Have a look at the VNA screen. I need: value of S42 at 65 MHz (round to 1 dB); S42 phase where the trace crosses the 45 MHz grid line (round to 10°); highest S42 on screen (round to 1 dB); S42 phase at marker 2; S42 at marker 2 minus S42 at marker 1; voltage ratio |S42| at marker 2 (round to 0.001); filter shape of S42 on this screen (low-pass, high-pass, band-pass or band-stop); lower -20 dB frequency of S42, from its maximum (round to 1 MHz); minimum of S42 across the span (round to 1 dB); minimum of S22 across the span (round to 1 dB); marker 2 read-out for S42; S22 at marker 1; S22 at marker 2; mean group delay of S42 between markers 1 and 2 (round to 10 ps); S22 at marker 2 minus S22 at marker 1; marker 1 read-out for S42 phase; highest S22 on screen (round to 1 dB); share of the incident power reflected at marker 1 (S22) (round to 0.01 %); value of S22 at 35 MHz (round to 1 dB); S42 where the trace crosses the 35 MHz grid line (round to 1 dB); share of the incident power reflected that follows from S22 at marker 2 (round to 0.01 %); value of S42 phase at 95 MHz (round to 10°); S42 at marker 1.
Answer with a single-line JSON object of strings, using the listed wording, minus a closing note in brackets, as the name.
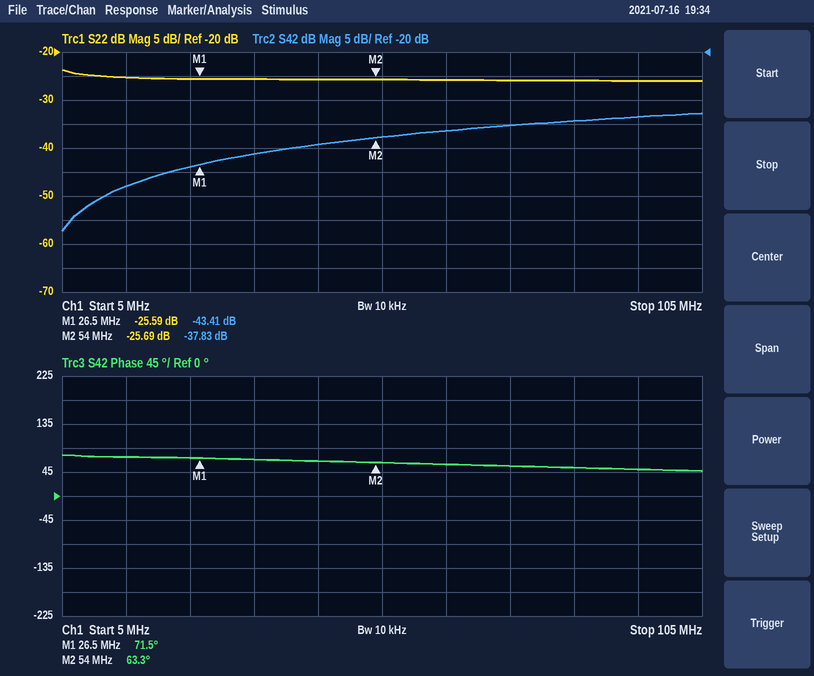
{"value of S42 at 65 MHz": "-36 dB", "S42 phase where the trace crosses the 45 MHz grid line": "70°", "highest S42 on screen": "-33 dB", "S42 phase at marker 2": "63.3°", "S42 at marker 2 minus S42 at marker 1": "5.58 dB", "voltage ratio |S42| at marker 2": "0.013", "filter shape of S42 on this screen": "high-pass", "lower -20 dB frequency of S42, from its maximum": "8 MHz", "minimum of S42 across the span": "-57 dB", "minimum of S22 across the span": "-26 dB", "marker 2 read-out for S42": "-37.83 dB", "S22 at marker 1": "-25.59 dB", "S22 at marker 2": "-25.69 dB", "mean group delay of S42 between markers 1 and 2": "830 ps", "S22 at marker 2 minus S22 at marker 1": "-0.10 dB", "marker 1 read-out for S42 phase": "71.5°", "highest S22 on screen": "-24 dB", "share of the incident power reflected at marker 1 (S22)": "0.28 %", "value of S22 at 35 MHz": "-26 dB", "S42 where the trace crosses the 35 MHz grid line": "-41 dB", "share of the incident power reflected that follows from S22 at marker 2": "0.27 %", "value of S42 phase at 95 MHz": "50°", "S42 at marker 1": "-43.41 dB"}
